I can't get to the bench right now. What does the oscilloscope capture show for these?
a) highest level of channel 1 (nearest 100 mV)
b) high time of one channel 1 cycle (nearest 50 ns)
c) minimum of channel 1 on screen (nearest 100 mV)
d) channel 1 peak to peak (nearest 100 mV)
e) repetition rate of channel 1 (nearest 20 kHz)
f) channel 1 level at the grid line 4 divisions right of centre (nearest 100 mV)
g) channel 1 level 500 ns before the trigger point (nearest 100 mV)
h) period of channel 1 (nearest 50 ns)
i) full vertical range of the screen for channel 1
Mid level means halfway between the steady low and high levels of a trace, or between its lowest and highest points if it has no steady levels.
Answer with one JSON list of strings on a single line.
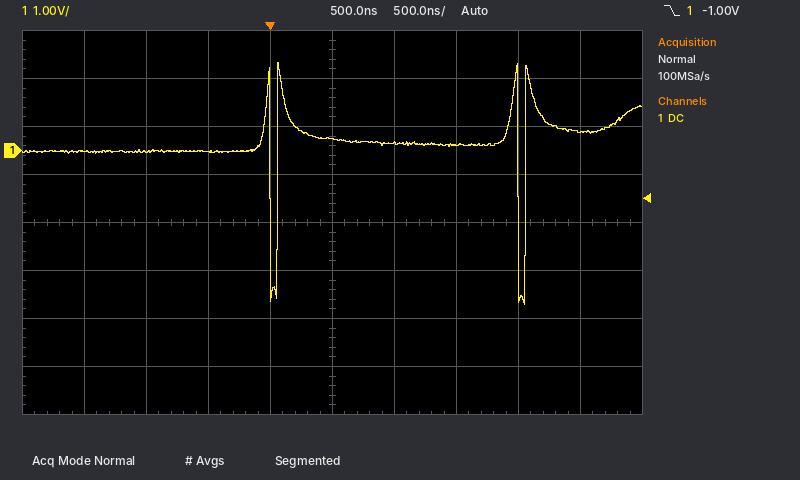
["1.8 V", "1.95 µs", "-3.2 V", "5.0 V", "500 kHz", "400 mV", "0.0 V", "2.00 µs", "8 V"]
